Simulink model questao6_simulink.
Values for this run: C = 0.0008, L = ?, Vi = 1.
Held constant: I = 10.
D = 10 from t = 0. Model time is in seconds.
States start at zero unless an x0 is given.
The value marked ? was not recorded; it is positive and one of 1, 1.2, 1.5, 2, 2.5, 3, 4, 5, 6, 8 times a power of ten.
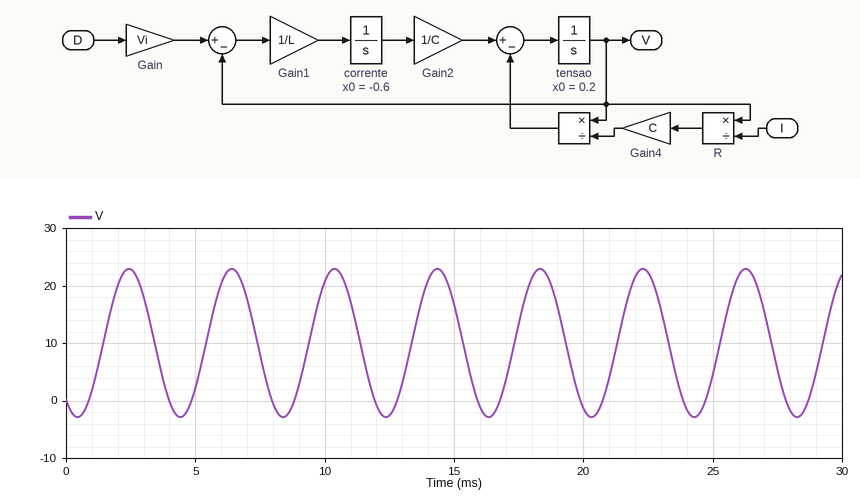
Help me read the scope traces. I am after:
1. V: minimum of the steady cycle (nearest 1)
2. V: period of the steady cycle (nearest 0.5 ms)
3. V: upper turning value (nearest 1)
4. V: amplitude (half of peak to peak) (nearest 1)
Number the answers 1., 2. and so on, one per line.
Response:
1. -3
2. 4.0 ms
3. 23
4. 13
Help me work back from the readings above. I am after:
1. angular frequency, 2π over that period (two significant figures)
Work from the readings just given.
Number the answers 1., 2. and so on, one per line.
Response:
1. 1.6 rad/ms
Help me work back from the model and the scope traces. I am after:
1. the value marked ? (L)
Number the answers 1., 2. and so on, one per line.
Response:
1. 0.0005
